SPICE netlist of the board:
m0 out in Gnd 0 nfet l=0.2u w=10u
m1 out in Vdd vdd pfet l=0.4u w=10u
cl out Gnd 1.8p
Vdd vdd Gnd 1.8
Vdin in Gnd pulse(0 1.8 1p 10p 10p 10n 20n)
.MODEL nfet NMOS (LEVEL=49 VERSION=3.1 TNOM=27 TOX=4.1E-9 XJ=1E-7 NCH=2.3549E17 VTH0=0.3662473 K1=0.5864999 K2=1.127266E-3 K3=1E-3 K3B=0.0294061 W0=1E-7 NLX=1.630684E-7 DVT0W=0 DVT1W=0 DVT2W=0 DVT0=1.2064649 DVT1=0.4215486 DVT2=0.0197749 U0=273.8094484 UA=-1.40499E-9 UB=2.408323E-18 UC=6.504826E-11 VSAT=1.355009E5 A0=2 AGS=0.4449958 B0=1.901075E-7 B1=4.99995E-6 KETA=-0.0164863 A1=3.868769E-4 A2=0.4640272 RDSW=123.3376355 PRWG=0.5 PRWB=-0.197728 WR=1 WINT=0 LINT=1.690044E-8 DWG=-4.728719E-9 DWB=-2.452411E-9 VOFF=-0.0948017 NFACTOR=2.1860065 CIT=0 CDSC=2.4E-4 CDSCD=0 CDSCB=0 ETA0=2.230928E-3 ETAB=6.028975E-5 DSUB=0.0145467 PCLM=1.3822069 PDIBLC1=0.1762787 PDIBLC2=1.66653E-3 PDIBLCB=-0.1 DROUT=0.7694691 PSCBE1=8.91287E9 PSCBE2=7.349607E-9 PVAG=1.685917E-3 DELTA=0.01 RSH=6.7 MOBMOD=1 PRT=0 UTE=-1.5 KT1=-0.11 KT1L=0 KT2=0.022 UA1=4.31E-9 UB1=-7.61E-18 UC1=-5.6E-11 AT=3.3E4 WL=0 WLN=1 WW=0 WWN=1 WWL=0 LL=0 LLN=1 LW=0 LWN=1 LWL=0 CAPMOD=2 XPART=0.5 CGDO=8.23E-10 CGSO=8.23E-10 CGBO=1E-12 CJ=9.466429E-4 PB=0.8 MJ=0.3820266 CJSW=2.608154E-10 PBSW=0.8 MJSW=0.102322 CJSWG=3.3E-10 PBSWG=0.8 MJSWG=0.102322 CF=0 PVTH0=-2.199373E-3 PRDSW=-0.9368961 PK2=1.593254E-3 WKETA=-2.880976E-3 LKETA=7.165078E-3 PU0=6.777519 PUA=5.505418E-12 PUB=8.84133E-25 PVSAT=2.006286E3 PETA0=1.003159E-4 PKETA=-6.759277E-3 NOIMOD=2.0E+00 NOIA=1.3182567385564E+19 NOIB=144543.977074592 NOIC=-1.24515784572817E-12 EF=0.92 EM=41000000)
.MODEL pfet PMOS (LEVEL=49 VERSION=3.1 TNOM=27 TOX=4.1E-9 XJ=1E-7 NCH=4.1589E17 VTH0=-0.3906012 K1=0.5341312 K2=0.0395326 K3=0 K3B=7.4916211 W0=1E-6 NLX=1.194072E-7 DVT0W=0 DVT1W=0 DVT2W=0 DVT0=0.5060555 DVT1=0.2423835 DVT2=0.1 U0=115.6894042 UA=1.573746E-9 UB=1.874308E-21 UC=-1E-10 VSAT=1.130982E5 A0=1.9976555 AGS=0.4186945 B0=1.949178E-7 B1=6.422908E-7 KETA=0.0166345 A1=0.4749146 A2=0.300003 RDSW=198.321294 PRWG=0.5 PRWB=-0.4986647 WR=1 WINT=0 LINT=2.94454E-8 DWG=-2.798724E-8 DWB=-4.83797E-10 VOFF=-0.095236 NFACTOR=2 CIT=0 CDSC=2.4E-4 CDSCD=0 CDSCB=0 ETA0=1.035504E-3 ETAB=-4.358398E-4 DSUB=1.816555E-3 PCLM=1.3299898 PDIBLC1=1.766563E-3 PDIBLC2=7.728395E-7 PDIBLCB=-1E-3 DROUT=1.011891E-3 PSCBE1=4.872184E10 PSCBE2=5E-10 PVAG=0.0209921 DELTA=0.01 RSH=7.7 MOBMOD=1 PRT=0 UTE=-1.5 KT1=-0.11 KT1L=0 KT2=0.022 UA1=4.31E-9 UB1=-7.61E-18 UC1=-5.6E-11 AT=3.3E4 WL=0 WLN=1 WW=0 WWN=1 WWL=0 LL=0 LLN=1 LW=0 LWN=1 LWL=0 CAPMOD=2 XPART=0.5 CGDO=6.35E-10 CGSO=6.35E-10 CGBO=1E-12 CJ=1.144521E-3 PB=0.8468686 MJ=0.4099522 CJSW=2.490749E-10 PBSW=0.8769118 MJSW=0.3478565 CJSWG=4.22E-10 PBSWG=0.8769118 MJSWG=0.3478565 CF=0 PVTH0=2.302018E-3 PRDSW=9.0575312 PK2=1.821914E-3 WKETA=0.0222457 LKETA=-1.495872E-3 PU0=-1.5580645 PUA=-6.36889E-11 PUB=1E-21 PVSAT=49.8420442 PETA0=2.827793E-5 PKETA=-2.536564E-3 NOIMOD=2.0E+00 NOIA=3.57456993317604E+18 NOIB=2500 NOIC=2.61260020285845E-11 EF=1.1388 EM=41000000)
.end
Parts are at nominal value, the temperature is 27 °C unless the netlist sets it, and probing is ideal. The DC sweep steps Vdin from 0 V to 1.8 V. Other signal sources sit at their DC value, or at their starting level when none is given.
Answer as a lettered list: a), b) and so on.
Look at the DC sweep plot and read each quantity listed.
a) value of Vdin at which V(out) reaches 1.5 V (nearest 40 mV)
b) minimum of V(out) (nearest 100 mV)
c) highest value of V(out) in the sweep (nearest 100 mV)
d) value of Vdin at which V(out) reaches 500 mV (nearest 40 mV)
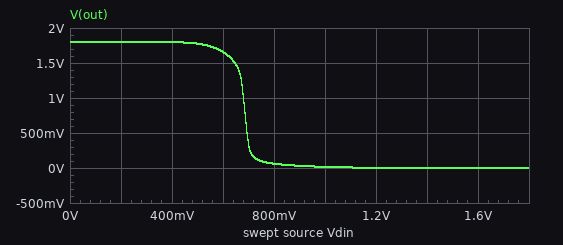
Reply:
a) 640 mV
b) 0 V
c) 1.8 V
d) 680 mV
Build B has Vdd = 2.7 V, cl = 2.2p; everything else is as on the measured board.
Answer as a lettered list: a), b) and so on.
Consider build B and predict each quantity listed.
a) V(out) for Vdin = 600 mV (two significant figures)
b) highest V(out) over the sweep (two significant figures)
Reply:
a) 2.6 V
b) 2.7 V
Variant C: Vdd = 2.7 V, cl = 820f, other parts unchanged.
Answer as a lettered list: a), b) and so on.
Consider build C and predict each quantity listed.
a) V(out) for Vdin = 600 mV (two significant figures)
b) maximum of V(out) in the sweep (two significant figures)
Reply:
a) 2.6 V
b) 2.7 V
